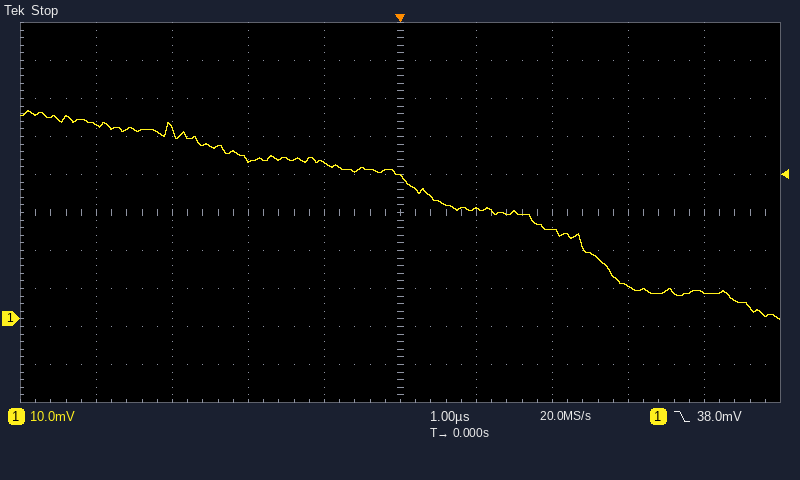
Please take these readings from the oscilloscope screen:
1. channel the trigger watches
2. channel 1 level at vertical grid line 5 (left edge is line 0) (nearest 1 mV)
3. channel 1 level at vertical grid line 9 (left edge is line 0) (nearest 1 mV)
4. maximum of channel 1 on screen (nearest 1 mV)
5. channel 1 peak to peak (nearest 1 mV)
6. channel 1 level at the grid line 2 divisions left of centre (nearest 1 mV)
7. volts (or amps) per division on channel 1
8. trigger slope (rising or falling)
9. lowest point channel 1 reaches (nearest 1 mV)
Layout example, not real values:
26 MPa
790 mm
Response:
channel 1
37 mV
7 mV
55 mV
55 mV
42 mV
10 mV
falling
0 mV
